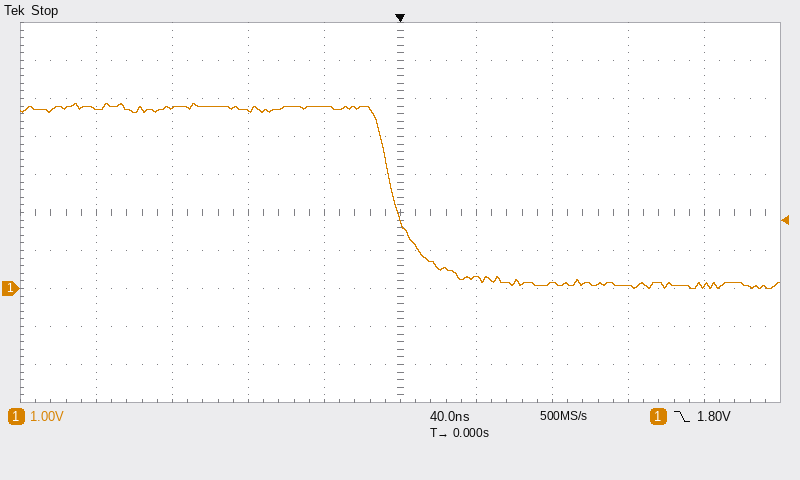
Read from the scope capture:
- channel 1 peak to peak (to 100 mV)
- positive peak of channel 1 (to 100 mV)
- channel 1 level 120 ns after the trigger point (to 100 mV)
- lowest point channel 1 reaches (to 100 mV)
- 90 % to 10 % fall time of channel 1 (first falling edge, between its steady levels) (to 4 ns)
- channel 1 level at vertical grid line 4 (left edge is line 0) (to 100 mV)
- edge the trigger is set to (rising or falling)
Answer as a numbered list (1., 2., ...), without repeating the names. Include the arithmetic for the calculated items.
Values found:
1. 4.9 V − (0.0 V) = 4.9 V
2. 4.9 V
3. 100 mV
4. 0.0 V
5. 32 ns
6. 4.8 V
7. falling
